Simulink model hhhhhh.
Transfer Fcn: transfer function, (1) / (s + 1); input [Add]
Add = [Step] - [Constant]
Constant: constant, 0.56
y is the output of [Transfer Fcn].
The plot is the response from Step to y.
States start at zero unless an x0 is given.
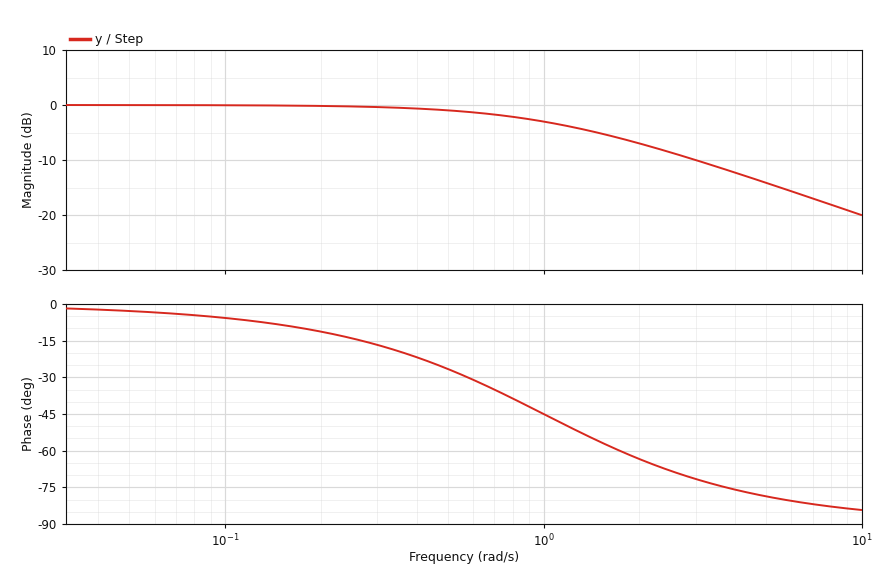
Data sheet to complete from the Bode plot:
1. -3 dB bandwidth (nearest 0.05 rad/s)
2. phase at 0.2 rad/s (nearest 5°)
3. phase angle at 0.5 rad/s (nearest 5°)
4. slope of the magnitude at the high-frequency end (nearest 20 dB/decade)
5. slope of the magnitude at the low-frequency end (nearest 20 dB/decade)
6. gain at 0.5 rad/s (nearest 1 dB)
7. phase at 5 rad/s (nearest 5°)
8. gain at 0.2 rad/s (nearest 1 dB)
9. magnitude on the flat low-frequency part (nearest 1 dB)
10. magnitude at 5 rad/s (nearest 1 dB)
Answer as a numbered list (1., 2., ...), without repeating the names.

1. 1.00 rad/s
2. -10°
3. -25°
4. -20 dB/decade
5. 0 dB/decade
6. -1 dB
7. -80°
8. 0 dB
9. 0 dB
10. -14 dB
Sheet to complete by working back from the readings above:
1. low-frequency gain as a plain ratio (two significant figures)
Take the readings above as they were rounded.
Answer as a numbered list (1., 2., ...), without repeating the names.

1. 1.0
